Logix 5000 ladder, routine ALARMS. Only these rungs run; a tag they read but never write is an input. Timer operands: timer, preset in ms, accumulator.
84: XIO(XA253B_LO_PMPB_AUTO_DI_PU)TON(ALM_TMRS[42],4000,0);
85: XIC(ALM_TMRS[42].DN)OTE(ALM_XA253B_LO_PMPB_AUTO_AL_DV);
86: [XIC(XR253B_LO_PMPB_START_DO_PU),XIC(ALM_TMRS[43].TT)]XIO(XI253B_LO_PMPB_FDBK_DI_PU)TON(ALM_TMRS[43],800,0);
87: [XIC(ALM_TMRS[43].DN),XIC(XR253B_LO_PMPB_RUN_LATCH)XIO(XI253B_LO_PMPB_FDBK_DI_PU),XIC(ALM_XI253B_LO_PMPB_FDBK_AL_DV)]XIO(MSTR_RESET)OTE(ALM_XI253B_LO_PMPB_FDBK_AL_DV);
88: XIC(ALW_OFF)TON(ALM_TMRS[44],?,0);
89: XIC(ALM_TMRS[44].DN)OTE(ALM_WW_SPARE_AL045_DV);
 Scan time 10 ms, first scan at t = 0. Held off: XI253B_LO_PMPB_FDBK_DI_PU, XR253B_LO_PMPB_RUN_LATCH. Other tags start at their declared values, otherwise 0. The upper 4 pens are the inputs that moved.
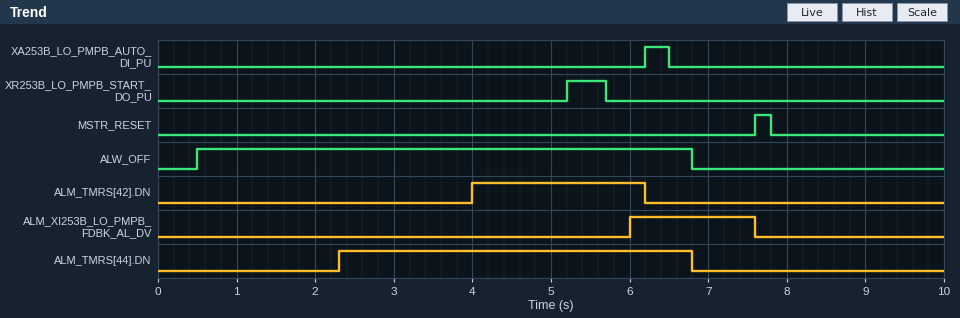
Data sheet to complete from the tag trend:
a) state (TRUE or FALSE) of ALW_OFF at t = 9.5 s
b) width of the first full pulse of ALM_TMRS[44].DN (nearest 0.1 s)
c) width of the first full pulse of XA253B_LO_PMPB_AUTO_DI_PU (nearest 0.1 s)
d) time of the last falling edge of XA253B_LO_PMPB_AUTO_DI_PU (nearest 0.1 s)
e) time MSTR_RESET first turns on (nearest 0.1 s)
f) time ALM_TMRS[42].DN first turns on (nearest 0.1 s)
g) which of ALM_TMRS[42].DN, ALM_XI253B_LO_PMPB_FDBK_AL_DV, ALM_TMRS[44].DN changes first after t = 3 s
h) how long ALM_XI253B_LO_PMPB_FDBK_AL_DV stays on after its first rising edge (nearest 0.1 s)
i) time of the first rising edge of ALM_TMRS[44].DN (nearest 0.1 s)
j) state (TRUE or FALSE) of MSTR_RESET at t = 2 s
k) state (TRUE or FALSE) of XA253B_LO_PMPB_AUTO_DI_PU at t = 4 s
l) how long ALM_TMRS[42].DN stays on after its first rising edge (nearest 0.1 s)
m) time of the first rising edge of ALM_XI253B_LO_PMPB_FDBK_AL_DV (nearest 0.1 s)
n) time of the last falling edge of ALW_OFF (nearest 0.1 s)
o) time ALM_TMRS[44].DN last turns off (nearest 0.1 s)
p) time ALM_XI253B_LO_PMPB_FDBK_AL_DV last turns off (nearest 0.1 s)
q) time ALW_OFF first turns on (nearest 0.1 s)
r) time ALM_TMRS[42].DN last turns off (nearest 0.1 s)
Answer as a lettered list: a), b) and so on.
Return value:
a) FALSE
b) 4.5 s
c) 0.3 s
d) 6.5 s
e) 7.6 s
f) 4.0 s
g) ALM_TMRS[42].DN
h) 1.6 s
i) 2.3 s
j) FALSE
k) FALSE
l) 2.2 s
m) 6.0 s
n) 6.8 s
o) 6.8 s
p) 7.6 s
q) 0.5 s
r) 6.2 s
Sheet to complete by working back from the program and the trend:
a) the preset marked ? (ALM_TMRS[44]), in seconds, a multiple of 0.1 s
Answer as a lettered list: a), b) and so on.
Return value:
a) 1.8 s
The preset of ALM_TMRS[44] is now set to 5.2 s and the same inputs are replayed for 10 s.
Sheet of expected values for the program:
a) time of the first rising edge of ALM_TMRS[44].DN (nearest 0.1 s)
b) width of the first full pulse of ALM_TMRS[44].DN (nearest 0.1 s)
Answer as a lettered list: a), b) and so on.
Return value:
a) 5.7 s
b) 1.1 s
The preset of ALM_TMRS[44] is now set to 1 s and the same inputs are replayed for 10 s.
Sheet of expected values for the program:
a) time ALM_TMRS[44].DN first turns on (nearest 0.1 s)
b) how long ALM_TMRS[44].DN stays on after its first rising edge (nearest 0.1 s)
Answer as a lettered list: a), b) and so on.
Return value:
a) 1.5 s
b) 5.3 s
